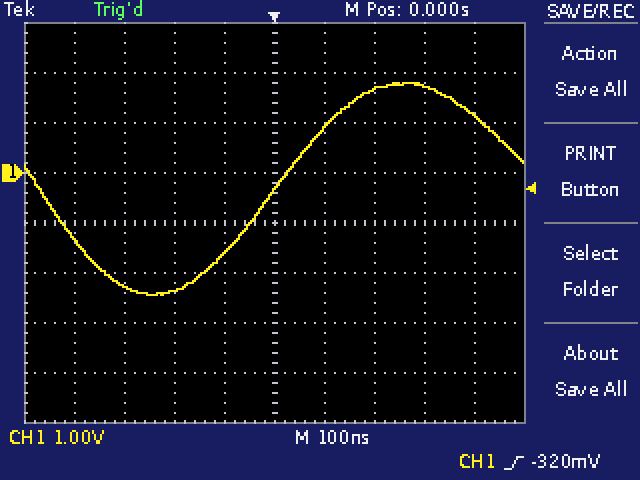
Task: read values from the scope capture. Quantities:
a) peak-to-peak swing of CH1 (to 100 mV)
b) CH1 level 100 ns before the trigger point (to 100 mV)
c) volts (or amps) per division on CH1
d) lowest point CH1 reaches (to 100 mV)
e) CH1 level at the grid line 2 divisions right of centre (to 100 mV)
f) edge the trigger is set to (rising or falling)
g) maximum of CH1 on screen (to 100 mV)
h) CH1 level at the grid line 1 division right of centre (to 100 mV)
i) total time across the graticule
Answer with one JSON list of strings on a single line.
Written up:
["4.2 V", "-1.6 V", "1 V", "-2.4 V", "1.7 V", "rising", "1.8 V", "900 mV", "1 µs"]
